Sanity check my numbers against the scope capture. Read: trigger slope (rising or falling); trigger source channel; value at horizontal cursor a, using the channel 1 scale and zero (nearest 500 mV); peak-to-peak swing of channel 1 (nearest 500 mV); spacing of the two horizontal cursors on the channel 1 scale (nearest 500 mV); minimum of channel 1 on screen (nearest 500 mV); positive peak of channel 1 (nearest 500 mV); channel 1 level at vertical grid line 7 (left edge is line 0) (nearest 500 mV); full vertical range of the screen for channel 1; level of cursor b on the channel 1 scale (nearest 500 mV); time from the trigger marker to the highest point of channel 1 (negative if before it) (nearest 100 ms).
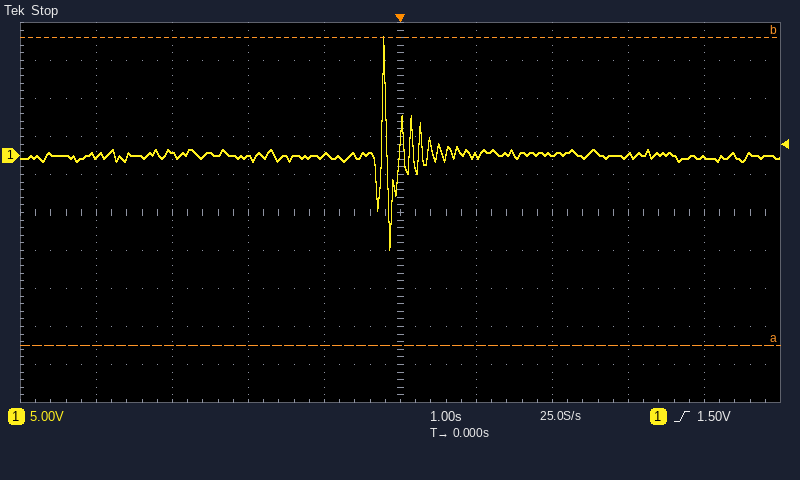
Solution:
rising
channel 1
-25.0 V
28.0 V
40.5 V
-12.5 V
15.5 V
0.0 V
50 V
15.5 V
-200 ms
